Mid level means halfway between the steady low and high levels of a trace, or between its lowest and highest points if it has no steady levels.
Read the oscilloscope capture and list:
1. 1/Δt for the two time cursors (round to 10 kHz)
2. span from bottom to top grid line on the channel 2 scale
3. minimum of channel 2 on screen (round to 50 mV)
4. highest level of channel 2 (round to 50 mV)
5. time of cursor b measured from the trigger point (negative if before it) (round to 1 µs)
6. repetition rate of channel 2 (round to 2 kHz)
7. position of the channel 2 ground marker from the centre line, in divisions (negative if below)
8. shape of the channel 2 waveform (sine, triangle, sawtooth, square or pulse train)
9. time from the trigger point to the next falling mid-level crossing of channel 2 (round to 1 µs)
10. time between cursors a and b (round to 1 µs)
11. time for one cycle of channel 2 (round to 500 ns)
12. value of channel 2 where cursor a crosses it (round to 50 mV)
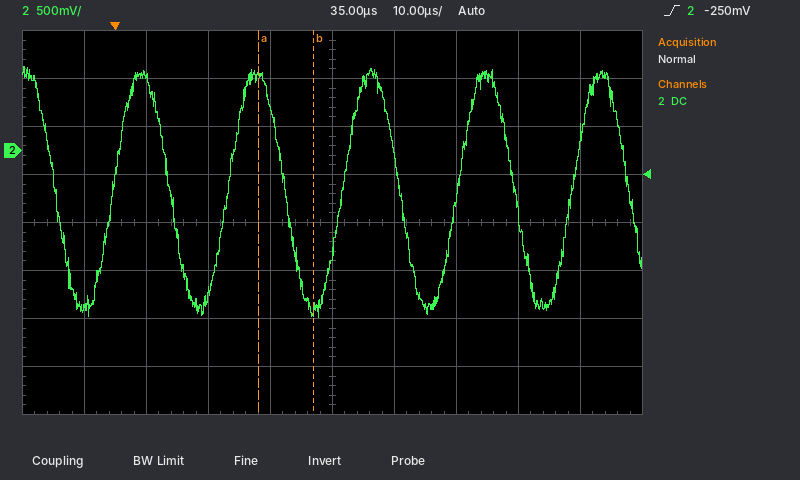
110 kHz
4 V
-1.75 V
900 mV
+32 µs
54 kHz
+1.5 div
sine
9 µs
9 µs
18.5 µs
750 mV
